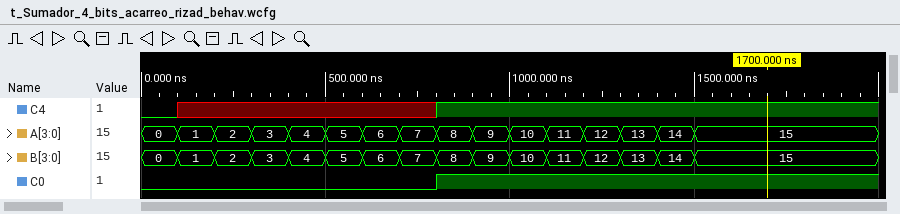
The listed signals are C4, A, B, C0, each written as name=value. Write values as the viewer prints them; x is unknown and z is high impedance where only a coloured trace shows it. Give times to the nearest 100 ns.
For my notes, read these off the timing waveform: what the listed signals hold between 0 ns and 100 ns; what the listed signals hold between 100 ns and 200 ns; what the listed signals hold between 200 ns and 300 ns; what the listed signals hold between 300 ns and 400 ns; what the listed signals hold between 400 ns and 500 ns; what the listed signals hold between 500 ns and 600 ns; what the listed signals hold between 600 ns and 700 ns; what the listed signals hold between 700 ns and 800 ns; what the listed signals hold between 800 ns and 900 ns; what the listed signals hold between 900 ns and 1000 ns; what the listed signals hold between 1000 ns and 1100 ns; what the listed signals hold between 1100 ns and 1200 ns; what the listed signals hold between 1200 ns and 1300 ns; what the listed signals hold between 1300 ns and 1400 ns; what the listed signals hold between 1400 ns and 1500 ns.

C4=0, A=0, B=0, C0=0
C4=x, A=1, B=1, C0=0
C4=x, A=2, B=2, C0=0
C4=x, A=3, B=3, C0=0
C4=x, A=4, B=4, C0=0
C4=x, A=5, B=5, C0=0
C4=x, A=6, B=6, C0=0
C4=x, A=7, B=7, C0=0
C4=1, A=8, B=8, C0=1
C4=1, A=9, B=9, C0=1
C4=1, A=10, B=10, C0=1
C4=1, A=11, B=11, C0=1
C4=1, A=12, B=12, C0=1
C4=1, A=13, B=13, C0=1
C4=1, A=14, B=14, C0=1
